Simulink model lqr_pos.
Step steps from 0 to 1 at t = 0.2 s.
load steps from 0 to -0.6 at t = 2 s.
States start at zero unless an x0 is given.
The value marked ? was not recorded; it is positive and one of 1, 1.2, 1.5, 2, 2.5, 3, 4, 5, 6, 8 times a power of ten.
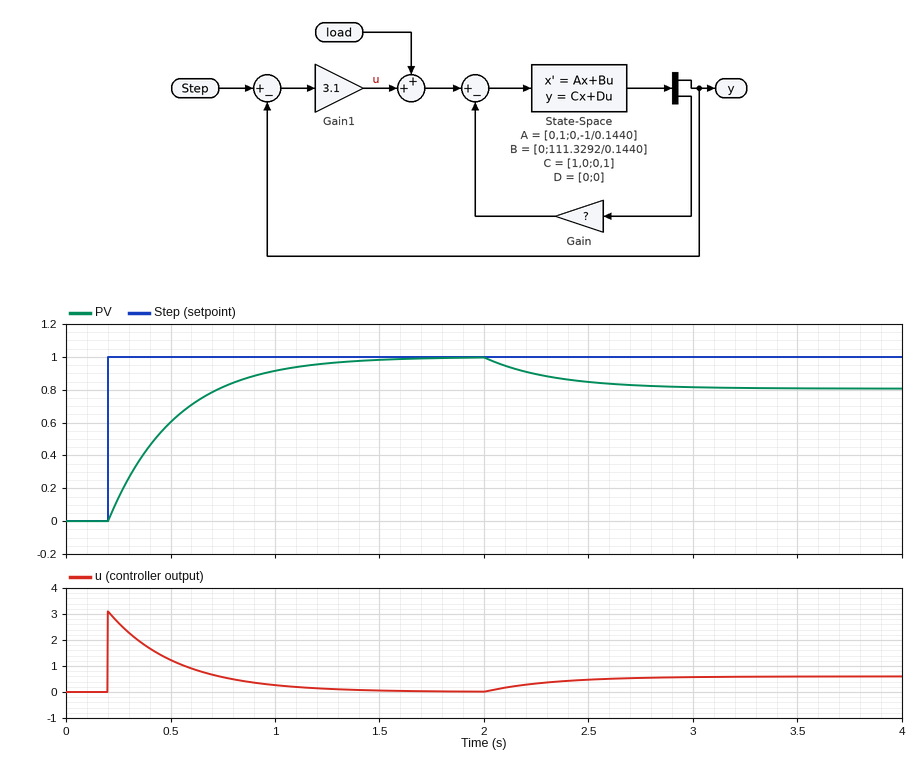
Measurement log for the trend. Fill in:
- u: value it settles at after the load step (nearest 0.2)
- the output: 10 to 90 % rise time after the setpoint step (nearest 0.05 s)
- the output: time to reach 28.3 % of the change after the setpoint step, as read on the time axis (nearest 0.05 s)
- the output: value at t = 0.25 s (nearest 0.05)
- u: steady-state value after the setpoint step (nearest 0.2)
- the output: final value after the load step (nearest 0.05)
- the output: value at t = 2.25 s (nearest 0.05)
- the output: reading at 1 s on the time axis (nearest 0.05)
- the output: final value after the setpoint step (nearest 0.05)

0.6
0.70 s
0.30 s
0.15
0.0
0.80
0.90
0.90
1.00
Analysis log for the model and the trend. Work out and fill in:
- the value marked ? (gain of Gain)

1
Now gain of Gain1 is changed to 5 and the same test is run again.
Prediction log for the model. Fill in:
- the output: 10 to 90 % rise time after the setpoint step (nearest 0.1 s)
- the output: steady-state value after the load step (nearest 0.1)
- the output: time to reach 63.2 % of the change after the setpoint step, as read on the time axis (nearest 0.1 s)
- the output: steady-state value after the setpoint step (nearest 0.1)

0.4 s
0.9
0.4 s
1.0
